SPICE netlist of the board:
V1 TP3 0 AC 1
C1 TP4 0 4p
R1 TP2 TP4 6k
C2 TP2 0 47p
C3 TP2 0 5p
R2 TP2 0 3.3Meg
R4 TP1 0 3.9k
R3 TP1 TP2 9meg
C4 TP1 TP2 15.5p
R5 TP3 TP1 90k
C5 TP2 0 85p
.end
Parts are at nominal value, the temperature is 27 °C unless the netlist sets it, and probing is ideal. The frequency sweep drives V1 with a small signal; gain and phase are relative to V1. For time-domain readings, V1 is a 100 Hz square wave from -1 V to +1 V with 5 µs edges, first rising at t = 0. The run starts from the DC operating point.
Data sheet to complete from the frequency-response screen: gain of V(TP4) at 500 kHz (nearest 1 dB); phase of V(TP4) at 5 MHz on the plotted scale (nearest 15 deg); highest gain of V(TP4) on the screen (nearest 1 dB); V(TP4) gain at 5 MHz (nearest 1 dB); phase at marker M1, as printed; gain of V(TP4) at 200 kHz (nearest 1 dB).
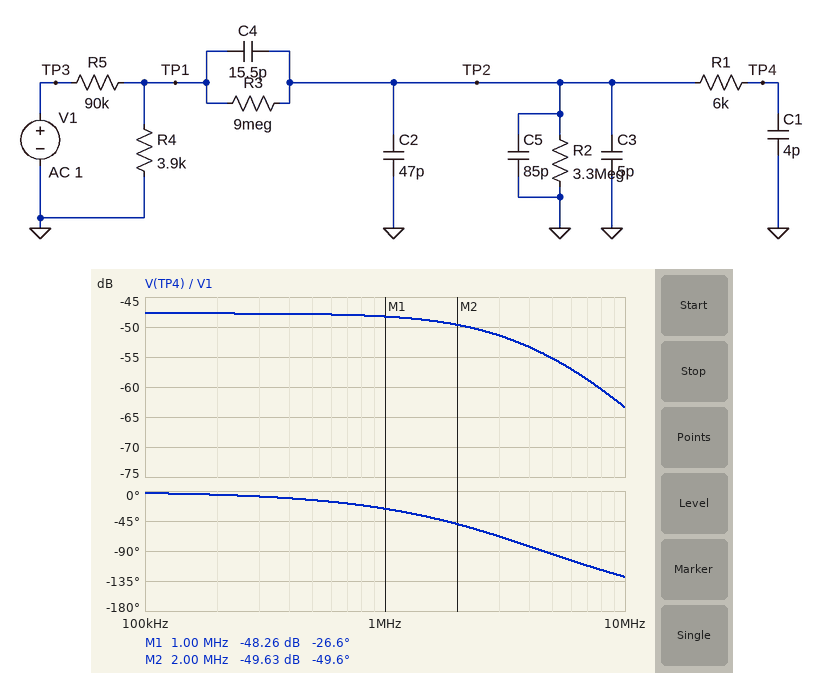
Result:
-48 dB
-90 deg
-48 dB
-55 dB
-26.6 deg
-48 dB
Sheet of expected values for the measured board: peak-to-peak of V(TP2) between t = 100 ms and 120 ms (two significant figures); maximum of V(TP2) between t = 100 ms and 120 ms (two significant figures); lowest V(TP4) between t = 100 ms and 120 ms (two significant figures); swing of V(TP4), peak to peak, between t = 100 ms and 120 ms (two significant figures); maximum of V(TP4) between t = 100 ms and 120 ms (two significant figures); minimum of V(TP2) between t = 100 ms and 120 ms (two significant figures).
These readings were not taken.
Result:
22 mV
11 mV
-11 mV
22 mV
11 mV
-11 mV
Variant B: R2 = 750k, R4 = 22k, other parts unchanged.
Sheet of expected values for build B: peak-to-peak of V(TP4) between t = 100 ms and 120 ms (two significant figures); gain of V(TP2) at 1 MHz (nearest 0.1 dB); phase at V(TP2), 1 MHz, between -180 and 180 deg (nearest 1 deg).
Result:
47 mV
-39.5 dB
-57 deg
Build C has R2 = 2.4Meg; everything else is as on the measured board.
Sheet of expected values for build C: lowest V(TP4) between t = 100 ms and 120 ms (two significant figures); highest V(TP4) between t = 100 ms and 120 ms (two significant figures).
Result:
-8.7 mV
8.7 mV
